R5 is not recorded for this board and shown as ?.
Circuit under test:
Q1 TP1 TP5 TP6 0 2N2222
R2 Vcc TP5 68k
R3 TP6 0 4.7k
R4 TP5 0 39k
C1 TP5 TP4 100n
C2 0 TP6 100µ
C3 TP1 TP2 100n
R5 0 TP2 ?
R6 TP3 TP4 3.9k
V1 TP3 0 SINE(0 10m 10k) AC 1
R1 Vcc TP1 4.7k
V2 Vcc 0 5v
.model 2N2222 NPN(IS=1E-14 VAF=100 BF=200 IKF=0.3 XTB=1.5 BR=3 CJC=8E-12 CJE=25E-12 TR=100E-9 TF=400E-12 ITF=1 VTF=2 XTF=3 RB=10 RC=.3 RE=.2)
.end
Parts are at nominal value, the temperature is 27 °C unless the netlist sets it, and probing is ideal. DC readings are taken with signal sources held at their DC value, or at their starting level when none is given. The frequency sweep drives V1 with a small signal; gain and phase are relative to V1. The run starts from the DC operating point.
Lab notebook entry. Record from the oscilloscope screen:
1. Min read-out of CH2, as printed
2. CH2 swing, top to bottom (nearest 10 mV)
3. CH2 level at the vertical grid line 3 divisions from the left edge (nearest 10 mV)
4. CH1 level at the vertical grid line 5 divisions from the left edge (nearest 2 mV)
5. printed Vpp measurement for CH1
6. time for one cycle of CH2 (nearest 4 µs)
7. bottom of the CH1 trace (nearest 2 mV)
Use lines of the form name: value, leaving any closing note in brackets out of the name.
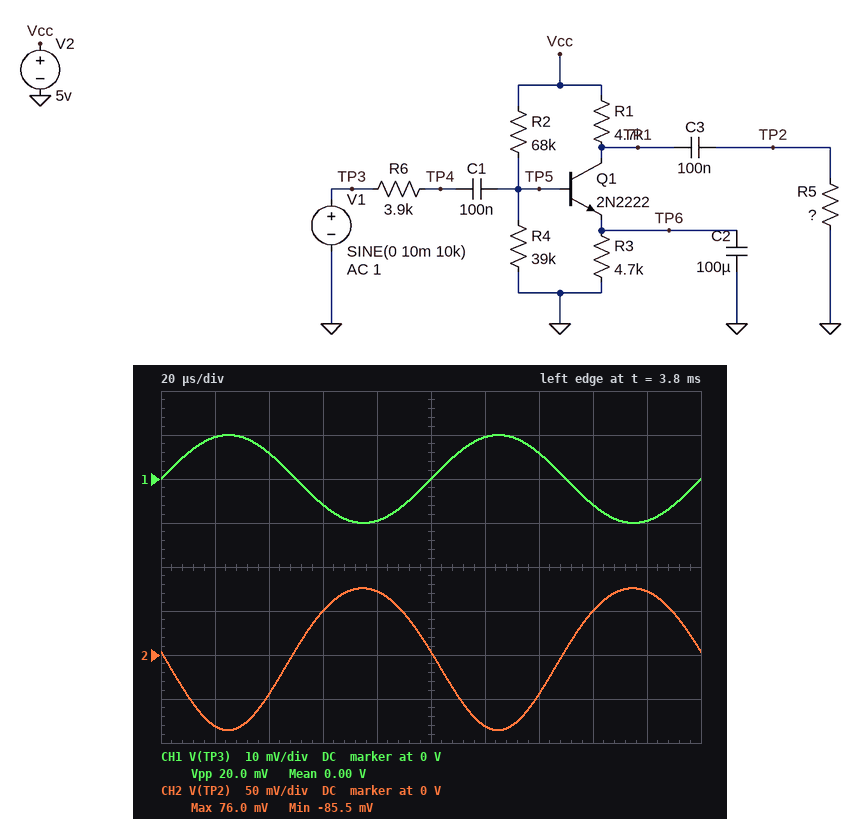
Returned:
Min read-out of CH2, as printed: -85.5 mV
CH2 swing, top to bottom: 160 mV
CH2 level at the vertical grid line 3 divisions from the left edge: 50 mV
CH1 level at the vertical grid line 5 divisions from the left edge: 0 V
printed Vpp measurement for CH1: 20.0 mV
time for one cycle of CH2: 100 µs
bottom of the CH1 trace: -10 mV
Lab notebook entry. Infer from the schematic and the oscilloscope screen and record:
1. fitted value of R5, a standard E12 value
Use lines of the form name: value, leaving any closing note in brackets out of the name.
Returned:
fitted value of R5, a standard E12 value: 1.5 kΩ
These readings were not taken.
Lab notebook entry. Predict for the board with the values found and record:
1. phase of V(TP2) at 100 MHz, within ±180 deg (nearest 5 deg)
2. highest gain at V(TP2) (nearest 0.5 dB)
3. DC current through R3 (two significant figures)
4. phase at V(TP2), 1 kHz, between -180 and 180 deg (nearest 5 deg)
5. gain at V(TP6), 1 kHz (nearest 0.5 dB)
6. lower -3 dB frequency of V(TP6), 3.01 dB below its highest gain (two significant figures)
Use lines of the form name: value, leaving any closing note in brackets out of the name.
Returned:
phase of V(TP2) at 100 MHz, within ±180 deg: 15 deg
highest gain at V(TP2): 18.0 dB
DC current through R3: 250 µA
phase at V(TP2), 1 kHz, between -180 and 180 deg: -160 deg
gain at V(TP6), 1 kHz: -39.0 dB
lower -3 dB frequency of V(TP6), 3.01 dB below its highest gain: 6.2 Hz
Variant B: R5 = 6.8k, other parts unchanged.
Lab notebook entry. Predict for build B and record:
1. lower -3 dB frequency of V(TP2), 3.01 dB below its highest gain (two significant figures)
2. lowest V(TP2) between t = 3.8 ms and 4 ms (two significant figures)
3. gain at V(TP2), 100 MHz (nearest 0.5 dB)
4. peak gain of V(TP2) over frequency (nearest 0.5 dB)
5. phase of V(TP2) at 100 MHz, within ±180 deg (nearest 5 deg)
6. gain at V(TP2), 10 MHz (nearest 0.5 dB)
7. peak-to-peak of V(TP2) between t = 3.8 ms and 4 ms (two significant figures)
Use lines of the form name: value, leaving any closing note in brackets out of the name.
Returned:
lower -3 dB frequency of V(TP2), 3.01 dB below its highest gain: 190 Hz
lowest V(TP2) between t = 3.8 ms and 4 ms: -210 mV
gain at V(TP2), 100 MHz: -31.5 dB
peak gain of V(TP2) over frequency: 26.0 dB
phase of V(TP2) at 100 MHz, within ±180 deg: 10 deg
gain at V(TP2), 10 MHz: -5.0 dB
peak-to-peak of V(TP2) between t = 3.8 ms and 4 ms: 390 mV
